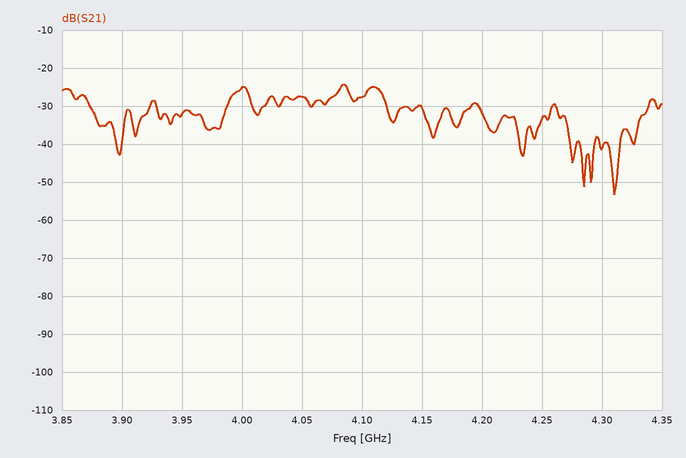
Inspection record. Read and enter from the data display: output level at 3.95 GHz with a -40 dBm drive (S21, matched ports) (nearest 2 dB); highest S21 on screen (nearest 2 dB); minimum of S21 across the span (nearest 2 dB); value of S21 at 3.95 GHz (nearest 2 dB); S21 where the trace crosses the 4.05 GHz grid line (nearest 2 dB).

-72 dBm
-24 dB
-54 dB
-32 dB
-28 dB
